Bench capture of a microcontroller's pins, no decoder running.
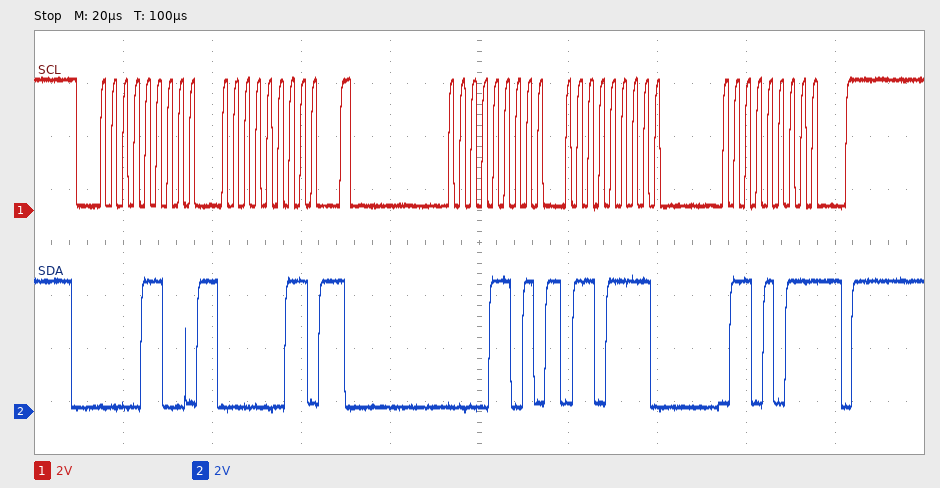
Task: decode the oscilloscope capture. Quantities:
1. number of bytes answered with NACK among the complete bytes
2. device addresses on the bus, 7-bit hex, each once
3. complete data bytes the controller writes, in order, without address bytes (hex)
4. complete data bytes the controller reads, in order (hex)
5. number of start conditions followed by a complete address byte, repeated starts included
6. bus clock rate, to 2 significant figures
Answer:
1
0x06
03
6F 6B
2
400 kHz
